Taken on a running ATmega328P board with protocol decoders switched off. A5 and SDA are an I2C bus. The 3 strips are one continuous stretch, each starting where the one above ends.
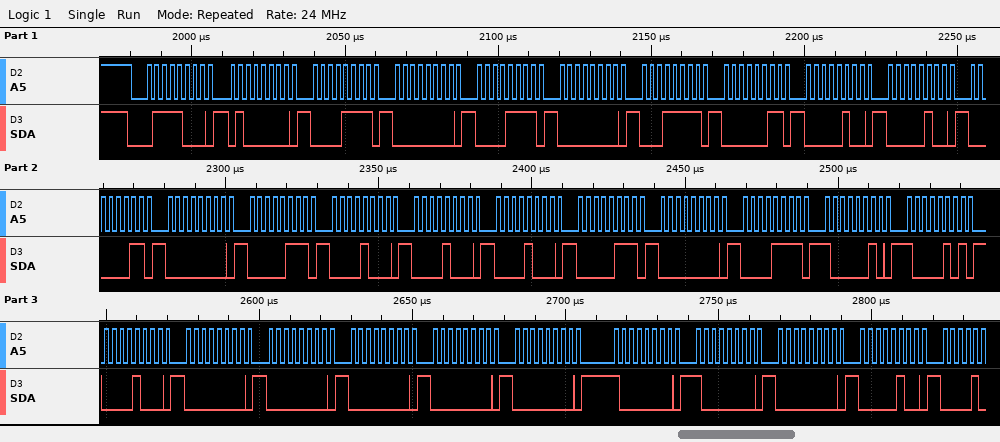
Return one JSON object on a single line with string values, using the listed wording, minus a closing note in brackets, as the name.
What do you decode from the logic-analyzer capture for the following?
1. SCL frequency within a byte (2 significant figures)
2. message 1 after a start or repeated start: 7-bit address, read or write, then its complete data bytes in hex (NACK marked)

{"SCL frequency within a byte": "400 kHz", "message 1 after a start or repeated start: 7-bit address, read or write, then its complete data bytes in hex": "0x3C write: 40 0F 00 0F 00 1F 03 04 04 03 00 07 08 08 08 07 00 0F 82 85 08 00 00 00 00 00 80 80 00 04"}
